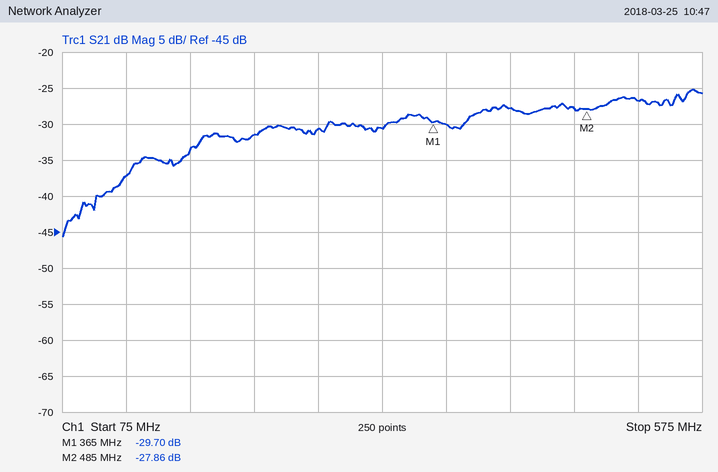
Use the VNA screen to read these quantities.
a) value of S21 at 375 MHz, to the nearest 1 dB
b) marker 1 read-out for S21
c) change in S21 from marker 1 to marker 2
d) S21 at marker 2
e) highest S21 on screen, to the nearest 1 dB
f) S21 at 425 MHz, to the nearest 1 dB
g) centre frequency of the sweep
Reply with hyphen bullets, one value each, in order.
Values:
- -30 dB
- -29.70 dB
- 1.84 dB
- -27.86 dB
- -25 dB
- -28 dB
- 325 MHz
